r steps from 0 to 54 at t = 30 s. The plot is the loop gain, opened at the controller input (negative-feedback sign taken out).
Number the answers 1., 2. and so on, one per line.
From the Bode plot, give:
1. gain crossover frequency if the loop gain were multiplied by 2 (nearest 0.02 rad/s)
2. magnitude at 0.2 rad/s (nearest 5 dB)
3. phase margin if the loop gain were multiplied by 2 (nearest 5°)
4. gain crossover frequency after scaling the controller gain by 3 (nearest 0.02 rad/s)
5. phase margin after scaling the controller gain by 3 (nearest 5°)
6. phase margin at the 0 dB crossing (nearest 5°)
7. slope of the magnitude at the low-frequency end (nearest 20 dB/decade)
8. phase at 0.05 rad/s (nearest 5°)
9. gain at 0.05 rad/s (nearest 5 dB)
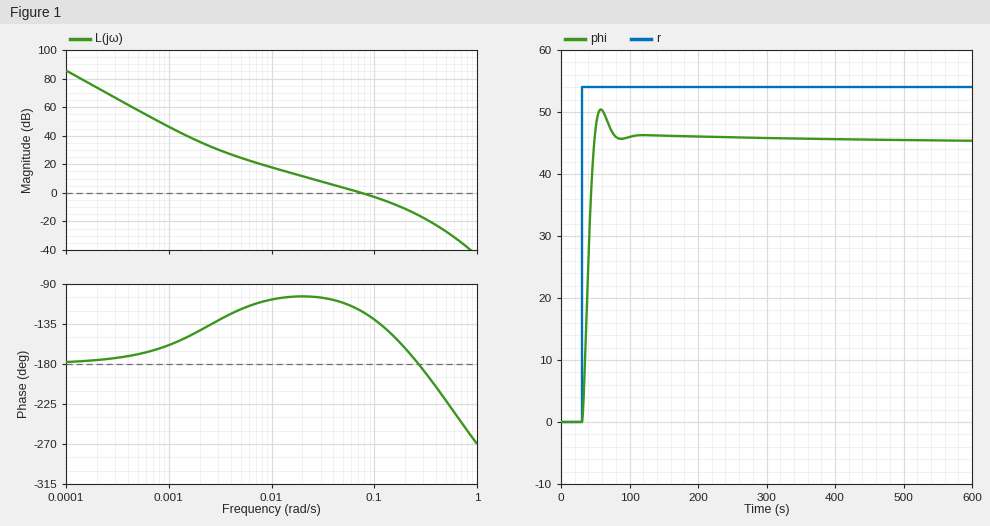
1. 0.14 rad/s
2. -10 dB
3. 40°
4. 0.18 rad/s
5. 25°
6. 60°
7. -40 dB/decade
8. -110°
9. 5 dB
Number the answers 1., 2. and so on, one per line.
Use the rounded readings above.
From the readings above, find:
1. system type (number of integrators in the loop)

1. 2
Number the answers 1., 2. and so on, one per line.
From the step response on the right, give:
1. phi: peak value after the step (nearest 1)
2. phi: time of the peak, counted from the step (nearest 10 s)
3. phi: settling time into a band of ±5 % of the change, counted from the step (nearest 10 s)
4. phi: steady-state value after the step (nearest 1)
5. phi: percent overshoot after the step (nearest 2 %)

1. 50
2. 30 s
3. 40 s
4. 45
5. 12 %
